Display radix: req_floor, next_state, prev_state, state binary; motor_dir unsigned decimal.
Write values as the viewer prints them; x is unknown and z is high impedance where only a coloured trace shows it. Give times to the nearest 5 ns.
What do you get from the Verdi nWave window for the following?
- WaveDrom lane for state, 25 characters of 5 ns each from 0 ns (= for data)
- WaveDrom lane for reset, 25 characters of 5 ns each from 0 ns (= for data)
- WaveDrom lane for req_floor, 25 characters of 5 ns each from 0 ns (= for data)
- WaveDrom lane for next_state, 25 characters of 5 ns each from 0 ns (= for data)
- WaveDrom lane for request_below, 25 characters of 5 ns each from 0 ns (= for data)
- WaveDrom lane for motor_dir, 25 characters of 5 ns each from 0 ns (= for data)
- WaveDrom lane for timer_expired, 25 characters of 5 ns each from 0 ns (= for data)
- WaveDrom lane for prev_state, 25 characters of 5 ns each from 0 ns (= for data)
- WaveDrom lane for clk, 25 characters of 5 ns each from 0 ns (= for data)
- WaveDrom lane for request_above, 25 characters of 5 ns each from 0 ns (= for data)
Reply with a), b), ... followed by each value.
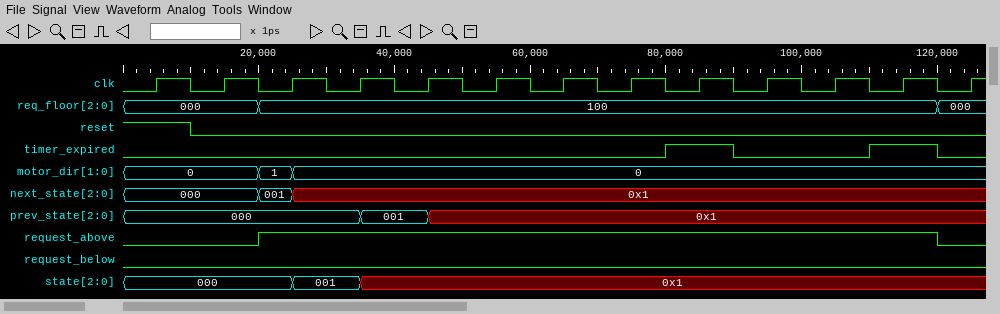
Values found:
a) {name: 'state', wave: '=....=.=.................', data: '000 001 0x1'}
b) {name: 'reset', wave: '1.0......................'}
c) {name: 'req_floor', wave: '=...=...................=', data: '000 100 000'}
d) {name: 'next_state', wave: '=...==...................', data: '000 001 0x1'}
e) {name: 'request_below', wave: '0........................'}
f) {name: 'motor_dir', wave: '=...==...................', data: '0 1 0'}
g) {name: 'timer_expired', wave: '0...............1.0...1.0'}
h) {name: 'prev_state', wave: '=......=.=...............', data: '000 001 0x1'}
i) {name: 'clk', wave: '0101010101010101010101010'}
j) {name: 'request_above', wave: '0...1...................0'}
